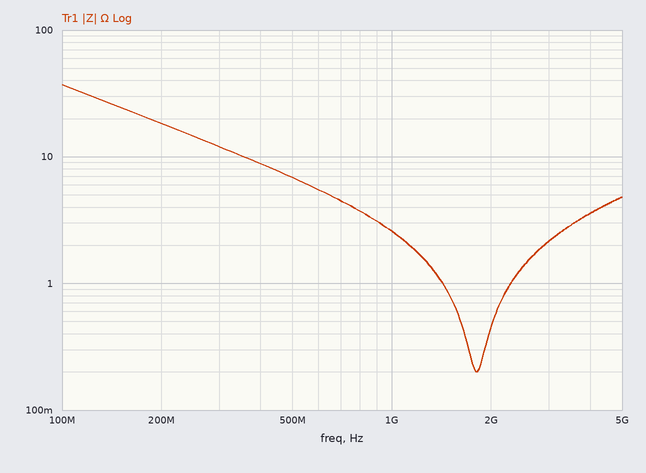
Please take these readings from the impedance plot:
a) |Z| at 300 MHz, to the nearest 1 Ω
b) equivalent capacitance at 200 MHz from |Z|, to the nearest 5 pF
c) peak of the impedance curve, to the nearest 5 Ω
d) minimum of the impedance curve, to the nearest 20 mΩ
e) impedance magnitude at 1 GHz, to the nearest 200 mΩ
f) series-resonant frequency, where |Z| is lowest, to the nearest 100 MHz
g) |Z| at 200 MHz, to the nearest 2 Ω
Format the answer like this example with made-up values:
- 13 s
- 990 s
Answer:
- 12 Ω
- 45 pF
- 35 Ω
- 200 mΩ
- 2.6 Ω
- 1.8 GHz
- 18 Ω
